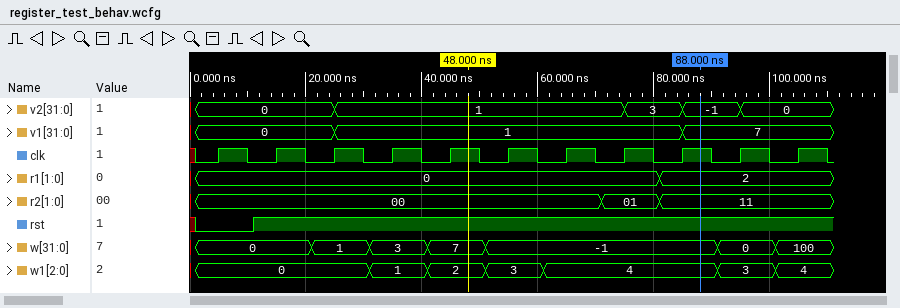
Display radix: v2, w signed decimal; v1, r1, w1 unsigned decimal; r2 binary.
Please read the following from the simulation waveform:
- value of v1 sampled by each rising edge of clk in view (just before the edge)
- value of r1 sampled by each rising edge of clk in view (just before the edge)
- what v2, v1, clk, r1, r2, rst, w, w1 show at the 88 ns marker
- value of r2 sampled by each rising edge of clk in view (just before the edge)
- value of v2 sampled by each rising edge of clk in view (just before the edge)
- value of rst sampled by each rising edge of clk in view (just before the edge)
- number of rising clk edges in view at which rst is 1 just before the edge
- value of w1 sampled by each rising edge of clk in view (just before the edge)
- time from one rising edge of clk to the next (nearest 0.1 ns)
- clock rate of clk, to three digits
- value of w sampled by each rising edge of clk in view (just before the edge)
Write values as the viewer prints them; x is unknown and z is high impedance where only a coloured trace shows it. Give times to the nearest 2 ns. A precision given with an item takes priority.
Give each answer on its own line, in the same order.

0, 0, 0, 1, 1, 1, 1, 1, 1, 7, 7
0, 0, 0, 0, 0, 0, 0, 0, 2, 2, 2
v2=-1, v1=7, clk=1, r1=2, r2=11, rst=1, w=-1, w1=4
00, 00, 00, 00, 00, 00, 00, 01, 11, 11, 11
0, 0, 0, 1, 1, 1, 1, 1, 3, -1, 0
0 1 1 1 1 1 1 1 1 1 1
10
0, 0, 0, 1, 2, 3, 4, 4, 4, 3, 4
10 ns
100 MHz
0, 0, 1, 3, 7, -1, -1, -1, -1, 0, 100
